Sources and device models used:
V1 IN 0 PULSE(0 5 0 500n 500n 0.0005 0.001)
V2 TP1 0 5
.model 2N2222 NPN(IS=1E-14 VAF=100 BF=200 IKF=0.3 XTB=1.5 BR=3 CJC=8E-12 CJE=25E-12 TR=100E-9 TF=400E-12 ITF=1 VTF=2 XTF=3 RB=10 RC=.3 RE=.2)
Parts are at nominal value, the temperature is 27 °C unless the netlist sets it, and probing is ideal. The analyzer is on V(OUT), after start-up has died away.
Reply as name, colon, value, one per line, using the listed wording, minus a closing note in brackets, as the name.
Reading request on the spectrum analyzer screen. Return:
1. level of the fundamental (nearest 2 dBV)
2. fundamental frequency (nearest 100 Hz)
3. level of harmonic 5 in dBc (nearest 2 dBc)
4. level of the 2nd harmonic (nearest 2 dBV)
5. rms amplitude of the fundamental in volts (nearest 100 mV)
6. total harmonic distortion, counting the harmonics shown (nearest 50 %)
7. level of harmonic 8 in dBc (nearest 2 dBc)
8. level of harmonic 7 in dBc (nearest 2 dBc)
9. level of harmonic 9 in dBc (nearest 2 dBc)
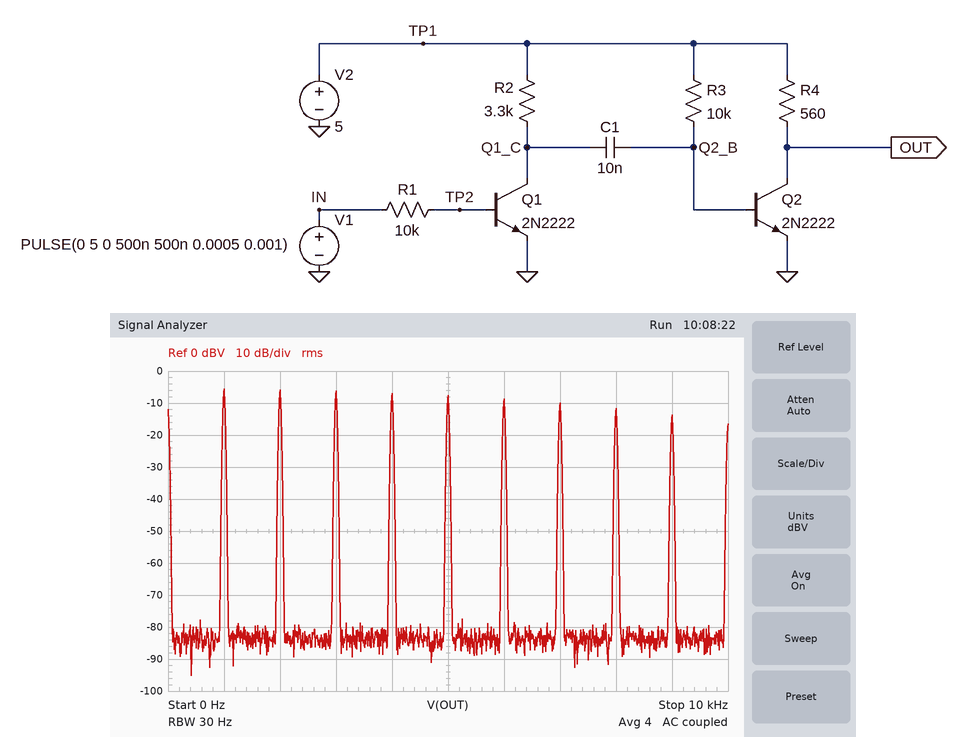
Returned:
level of the fundamental: -6 dBV
fundamental frequency: 1.0 kHz
level of harmonic 5 in dBc: -2 dBc
level of the 2nd harmonic: -6 dBV
rms amplitude of the fundamental in volts: 500 mV
total harmonic distortion, counting the harmonics shown: 200 %
level of harmonic 8 in dBc: -6 dBc
level of harmonic 7 in dBc: -4 dBc
level of harmonic 9 in dBc: -8 dBc
